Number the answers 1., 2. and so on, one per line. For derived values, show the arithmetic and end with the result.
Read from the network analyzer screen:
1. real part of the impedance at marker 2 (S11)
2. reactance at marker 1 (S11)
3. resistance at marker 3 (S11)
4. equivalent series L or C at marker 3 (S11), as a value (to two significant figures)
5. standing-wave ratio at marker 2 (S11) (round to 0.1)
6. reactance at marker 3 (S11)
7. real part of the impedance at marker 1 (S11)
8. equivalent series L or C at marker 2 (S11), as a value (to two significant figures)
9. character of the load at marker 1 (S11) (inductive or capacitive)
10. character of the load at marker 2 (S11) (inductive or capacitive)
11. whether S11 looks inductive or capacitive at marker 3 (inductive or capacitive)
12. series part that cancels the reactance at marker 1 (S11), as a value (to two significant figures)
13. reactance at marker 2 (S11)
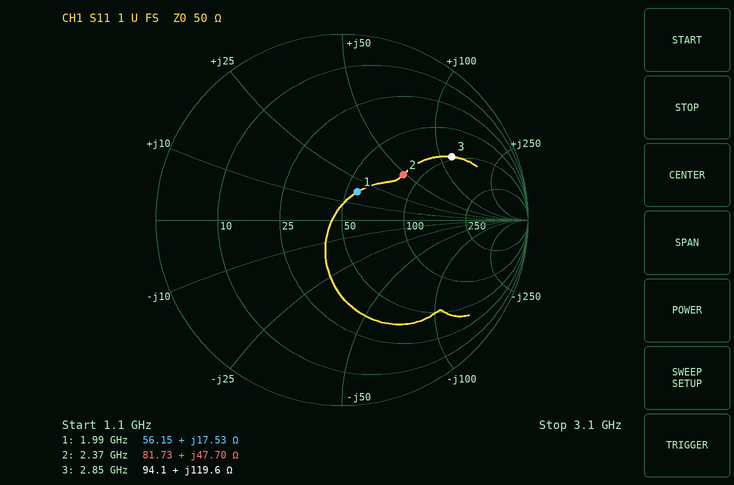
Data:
1. 81.73 Ω
2. +17.53 Ω
3. 94.1 Ω
4. L = 119.6 Ω/(2π × 2.85 GHz) ≈ 6.7 nH
5. 2.4
6. +119.6 Ω
7. 56.15 Ω
8. L = 47.7 Ω/(2π × 2.37 GHz) ≈ 3.2 nH
9. inductive
10. inductive
11. inductive
12. C = 1/(2π × 1.99 GHz × 17.53 Ω) ≈ 4.6 pF
13. +47.70 Ω
